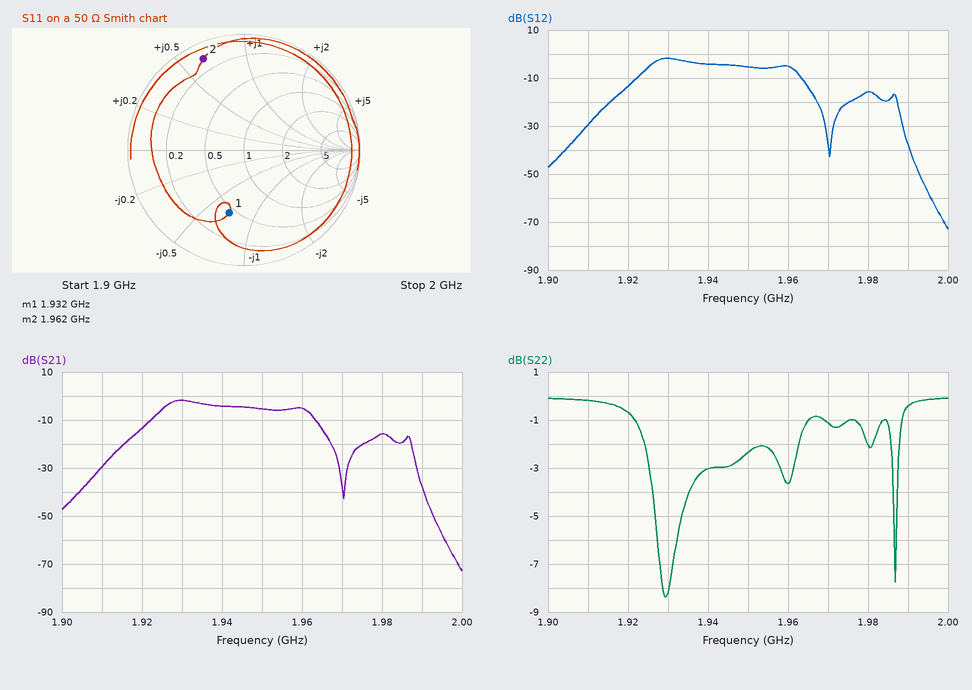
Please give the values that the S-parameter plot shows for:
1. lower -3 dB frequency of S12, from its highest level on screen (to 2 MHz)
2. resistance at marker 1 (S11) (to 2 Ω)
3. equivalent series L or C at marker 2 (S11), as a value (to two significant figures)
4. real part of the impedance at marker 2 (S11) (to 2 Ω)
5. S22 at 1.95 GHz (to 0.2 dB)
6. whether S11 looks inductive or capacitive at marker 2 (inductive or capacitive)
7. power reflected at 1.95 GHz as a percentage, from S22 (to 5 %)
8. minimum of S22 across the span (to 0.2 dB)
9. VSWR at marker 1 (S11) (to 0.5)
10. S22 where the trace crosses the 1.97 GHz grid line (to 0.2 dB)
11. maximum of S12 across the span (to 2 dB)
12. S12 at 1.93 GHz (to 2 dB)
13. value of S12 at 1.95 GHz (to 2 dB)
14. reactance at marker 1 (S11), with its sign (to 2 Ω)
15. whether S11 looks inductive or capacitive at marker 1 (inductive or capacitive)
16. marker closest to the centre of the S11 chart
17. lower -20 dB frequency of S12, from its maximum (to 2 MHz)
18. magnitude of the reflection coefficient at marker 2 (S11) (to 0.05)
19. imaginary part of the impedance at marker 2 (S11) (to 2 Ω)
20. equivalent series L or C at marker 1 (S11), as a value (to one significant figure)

1.926 GHz
22 Ω
2.6 nH
6 Ω
-2.4 dB
inductive
60 %
-8.4 dB
3.5
-1.2 dB
-2 dB
-2 dB
-6 dB
-34 Ω
capacitive
marker 1
1.914 GHz
0.85
+32 Ω
2 pF
